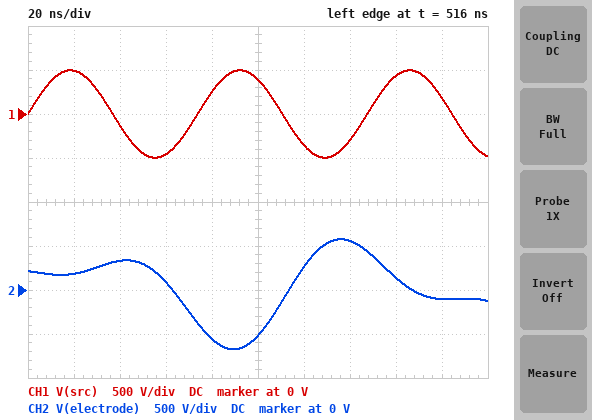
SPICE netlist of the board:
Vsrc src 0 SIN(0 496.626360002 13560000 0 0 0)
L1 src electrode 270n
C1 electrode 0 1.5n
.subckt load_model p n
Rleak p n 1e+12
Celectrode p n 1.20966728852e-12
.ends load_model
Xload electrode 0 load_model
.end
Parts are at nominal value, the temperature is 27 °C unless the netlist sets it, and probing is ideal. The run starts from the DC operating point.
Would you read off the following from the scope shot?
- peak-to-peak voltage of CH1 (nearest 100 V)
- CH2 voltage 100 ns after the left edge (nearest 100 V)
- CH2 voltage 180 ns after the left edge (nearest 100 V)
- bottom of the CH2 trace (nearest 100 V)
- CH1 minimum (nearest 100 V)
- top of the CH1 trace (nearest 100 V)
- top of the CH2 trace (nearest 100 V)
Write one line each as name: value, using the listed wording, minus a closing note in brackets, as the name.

peak-to-peak voltage of CH1: 1.0 kV
CH2 voltage 100 ns after the left edge: -500 V
CH2 voltage 180 ns after the left edge: -100 V
bottom of the CH2 trace: -700 V
CH1 minimum: -500 V
top of the CH1 trace: 500 V
top of the CH2 trace: 600 V
